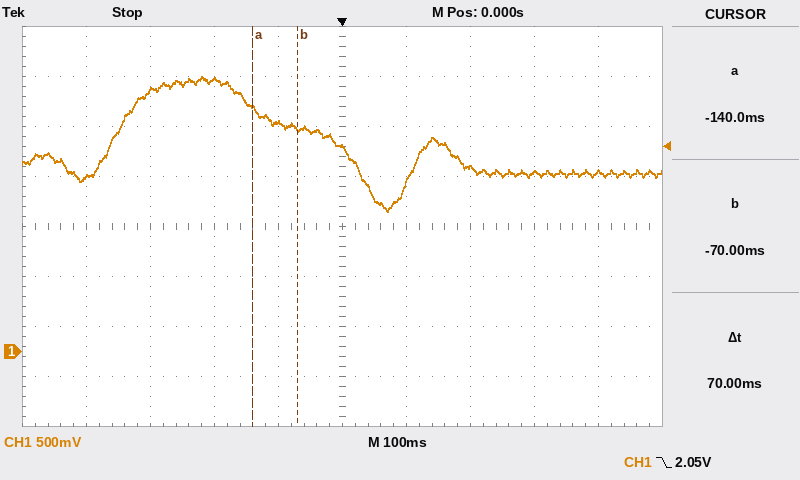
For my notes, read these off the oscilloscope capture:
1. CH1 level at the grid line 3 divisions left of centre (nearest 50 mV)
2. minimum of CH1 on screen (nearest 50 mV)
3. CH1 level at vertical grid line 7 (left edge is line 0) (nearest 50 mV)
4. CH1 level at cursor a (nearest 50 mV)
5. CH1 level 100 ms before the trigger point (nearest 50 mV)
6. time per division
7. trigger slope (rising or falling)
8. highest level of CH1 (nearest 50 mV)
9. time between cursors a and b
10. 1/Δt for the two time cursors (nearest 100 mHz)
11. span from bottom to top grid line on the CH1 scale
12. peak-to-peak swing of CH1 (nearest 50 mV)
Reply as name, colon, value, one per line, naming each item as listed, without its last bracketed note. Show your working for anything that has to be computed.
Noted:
CH1 level at the grid line 3 divisions left of centre: 2.60 V
minimum of CH1 on screen: 1.40 V
CH1 level at vertical grid line 7 (left edge is line 0): 1.85 V
CH1 level at cursor a: 2.45 V
CH1 level 100 ms before the trigger point: 2.30 V
time per division: 100 ms
trigger slope: falling
highest level of CH1: 2.75 V
time between cursors a and b: 70 ms
1/Δt for the two time cursors: 1 / 70 ms ≈ 14.3 Hz
span from bottom to top grid line on the CH1 scale: 4 V
peak-to-peak swing of CH1: 2.75 V − (1.40 V) = 1.35 V
